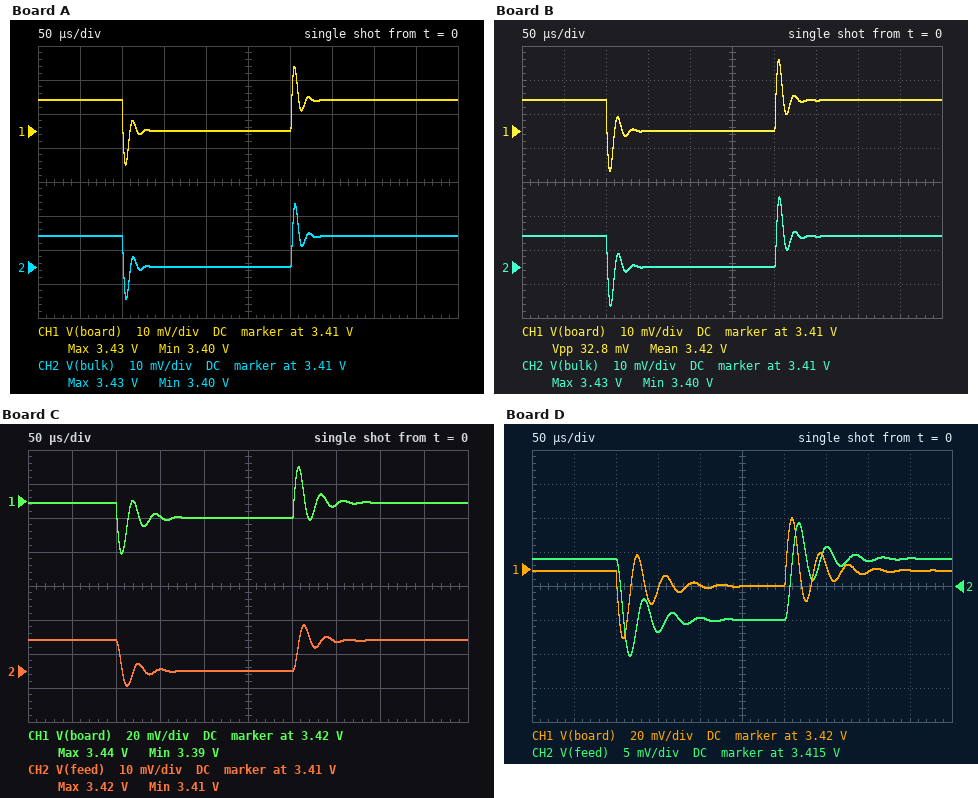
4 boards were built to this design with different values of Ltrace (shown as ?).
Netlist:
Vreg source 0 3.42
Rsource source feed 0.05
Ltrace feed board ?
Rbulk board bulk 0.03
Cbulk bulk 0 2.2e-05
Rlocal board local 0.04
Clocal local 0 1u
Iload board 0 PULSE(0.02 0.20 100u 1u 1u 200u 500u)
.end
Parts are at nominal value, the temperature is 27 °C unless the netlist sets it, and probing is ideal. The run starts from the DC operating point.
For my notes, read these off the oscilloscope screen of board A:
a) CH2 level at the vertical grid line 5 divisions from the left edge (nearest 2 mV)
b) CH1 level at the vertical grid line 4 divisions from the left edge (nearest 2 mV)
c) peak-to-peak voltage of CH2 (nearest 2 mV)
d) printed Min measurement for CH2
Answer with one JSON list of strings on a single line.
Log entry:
["3.410 V", "3.410 V", "28 mV", "3.40 V"]
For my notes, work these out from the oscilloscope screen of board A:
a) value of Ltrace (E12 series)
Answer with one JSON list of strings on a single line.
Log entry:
["270 nH"]
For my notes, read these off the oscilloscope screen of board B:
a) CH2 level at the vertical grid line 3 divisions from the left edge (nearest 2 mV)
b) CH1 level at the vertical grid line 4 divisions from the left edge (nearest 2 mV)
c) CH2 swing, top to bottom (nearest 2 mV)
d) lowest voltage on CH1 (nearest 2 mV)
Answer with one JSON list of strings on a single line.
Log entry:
["3.410 V", "3.410 V", "32 mV", "3.398 V"]
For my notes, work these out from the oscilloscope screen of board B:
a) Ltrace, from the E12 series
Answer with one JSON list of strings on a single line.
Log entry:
["330 nH"]
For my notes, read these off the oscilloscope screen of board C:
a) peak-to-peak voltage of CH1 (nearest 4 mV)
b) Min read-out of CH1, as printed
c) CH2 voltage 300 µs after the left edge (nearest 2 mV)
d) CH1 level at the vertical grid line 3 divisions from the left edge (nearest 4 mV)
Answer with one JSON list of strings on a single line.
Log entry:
["52 mV", "3.39 V", "3.410 V", "3.412 V"]
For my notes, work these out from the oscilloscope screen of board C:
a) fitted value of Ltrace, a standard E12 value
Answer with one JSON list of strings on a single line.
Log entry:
["680 nH"]
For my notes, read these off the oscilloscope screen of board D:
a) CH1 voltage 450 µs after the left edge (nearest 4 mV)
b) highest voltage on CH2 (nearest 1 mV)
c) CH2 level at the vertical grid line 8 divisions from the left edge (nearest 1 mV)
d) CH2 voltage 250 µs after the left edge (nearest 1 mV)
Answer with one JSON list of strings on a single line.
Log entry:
["3.420 V", "3.424 V", "3.419 V", "3.410 V"]
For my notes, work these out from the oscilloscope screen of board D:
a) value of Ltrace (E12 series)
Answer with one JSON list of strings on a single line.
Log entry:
["1.2 µH"]
